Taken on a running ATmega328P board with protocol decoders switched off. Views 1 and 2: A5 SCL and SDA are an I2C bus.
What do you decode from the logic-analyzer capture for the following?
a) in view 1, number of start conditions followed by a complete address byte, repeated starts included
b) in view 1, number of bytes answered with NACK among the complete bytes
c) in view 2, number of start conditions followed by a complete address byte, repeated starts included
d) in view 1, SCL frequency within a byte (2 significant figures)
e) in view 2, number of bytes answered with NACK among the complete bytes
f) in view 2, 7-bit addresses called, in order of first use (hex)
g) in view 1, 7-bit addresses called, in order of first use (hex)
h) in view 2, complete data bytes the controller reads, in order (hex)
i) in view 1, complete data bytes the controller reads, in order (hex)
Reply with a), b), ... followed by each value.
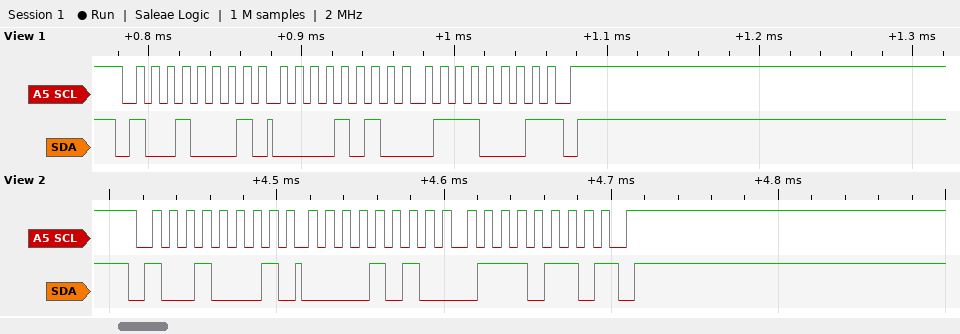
a) 1
b) 1
c) 1
d) 100 kHz
e) 1
f) 0x48
g) 0x48
h) 0A 76
i) 0A 71
